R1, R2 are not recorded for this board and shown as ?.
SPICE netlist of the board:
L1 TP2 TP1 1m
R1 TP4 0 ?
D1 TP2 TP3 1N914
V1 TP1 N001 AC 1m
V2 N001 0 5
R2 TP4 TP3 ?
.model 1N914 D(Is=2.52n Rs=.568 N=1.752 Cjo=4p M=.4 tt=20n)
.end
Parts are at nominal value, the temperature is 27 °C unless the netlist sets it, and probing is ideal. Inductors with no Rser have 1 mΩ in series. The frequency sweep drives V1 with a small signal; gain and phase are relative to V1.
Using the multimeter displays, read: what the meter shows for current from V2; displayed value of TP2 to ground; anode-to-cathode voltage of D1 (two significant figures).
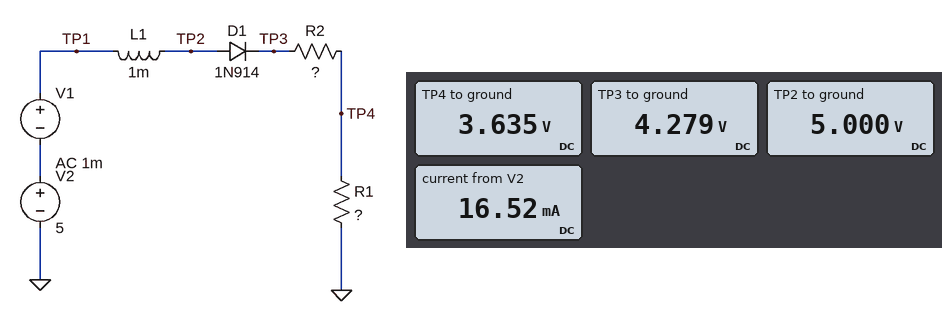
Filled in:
16.52 mA
5.000 V
720 mV
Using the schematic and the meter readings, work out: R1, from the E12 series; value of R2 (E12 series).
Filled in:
220 Ω
39 Ω
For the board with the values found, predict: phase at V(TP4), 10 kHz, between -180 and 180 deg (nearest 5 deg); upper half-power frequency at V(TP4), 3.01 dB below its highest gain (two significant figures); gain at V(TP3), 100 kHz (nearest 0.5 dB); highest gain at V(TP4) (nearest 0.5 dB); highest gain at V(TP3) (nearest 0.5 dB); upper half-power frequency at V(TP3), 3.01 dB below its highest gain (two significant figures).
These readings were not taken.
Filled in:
-15 deg
42 kHz
-8.5 dB
-1.5 dB
0 dB
42 kHz
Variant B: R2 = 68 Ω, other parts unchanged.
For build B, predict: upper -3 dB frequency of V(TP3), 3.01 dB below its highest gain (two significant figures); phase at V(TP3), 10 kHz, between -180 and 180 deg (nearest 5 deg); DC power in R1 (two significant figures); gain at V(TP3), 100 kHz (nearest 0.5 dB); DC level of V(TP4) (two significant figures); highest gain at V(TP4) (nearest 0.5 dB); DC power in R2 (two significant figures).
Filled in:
46 kHz
-10 deg
49 mW
-7.5 dB
3.3 V
-2.5 dB
15 mW
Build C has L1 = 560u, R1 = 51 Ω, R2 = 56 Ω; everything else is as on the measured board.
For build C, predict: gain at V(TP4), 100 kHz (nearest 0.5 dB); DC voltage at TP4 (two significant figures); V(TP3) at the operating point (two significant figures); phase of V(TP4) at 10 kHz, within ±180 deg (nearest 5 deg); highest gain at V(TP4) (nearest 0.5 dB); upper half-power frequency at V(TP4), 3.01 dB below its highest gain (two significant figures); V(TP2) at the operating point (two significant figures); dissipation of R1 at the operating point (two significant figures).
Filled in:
-17.0 dB
2.0 V
4.2 V
-20 deg
-6.5 dB
31 kHz
5.0 V
80 mW
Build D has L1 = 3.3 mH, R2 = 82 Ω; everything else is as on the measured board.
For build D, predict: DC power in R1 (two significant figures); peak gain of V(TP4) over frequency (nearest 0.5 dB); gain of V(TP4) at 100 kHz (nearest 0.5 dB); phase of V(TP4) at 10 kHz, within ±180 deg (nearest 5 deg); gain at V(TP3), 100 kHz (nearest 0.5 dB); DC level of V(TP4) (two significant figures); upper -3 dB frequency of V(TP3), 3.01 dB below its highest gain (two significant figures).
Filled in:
44 mW
-3.0 dB
-19.5 dB
-35 deg
-17.0 dB
3.1 V
15 kHz
